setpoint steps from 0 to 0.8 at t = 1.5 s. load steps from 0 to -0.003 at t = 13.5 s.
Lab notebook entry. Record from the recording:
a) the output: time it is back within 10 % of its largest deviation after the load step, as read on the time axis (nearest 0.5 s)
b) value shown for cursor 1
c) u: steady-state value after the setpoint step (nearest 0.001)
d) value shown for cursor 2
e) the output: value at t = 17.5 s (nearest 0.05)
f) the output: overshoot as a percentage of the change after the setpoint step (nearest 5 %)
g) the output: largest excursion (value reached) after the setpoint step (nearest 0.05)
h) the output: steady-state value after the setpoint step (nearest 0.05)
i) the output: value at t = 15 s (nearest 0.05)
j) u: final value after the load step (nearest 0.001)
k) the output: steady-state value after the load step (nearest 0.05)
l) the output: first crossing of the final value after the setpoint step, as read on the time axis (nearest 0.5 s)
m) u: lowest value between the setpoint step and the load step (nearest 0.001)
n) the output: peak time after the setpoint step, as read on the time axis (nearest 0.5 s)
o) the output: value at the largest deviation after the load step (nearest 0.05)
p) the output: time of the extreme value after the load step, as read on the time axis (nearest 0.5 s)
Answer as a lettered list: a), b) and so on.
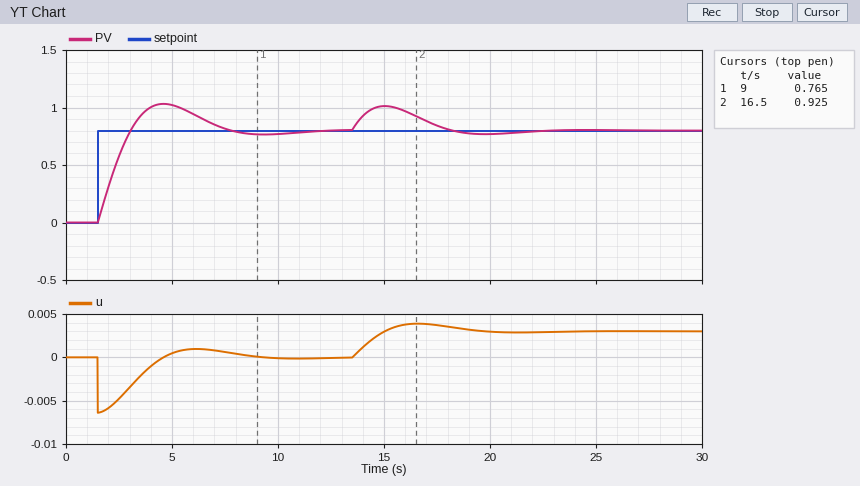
a) 21.0 s
b) 0.765
c) 0.000
d) 0.925
e) 0.85
f) 30 %
g) 1.05
h) 0.80
i) 1.00
j) 0.003
k) 0.80
l) 3.0 s
m) -0.006
n) 4.5 s
o) 1.00
p) 15.0 s
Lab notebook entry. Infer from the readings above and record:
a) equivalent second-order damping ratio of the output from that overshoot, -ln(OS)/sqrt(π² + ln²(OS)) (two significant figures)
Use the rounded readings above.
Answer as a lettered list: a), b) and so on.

a) 0.36
